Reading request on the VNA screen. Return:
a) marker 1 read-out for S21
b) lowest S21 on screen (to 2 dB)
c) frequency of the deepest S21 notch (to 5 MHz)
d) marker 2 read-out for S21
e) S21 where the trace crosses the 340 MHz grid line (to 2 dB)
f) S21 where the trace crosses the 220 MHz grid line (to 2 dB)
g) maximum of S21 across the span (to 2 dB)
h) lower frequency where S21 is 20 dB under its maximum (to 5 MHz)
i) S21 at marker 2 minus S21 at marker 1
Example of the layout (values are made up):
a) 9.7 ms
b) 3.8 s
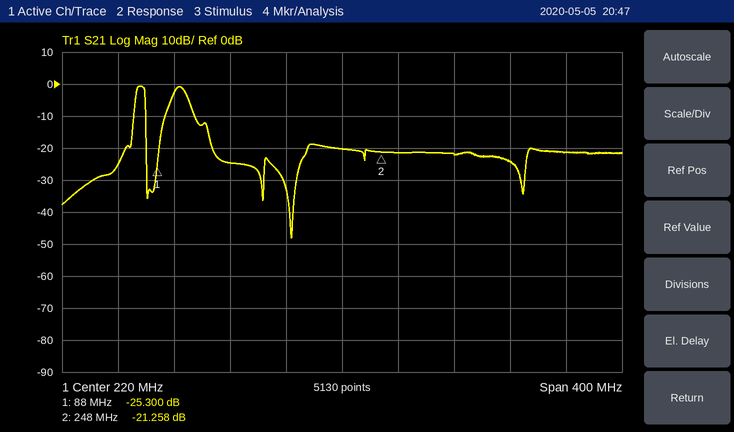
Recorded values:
a) -25.300 dB
b) -48 dB
c) 185 MHz
d) -21.258 dB
e) -24 dB
f) -20 dB
g) 0 dB
h) 65 MHz
i) 4.042 dB
